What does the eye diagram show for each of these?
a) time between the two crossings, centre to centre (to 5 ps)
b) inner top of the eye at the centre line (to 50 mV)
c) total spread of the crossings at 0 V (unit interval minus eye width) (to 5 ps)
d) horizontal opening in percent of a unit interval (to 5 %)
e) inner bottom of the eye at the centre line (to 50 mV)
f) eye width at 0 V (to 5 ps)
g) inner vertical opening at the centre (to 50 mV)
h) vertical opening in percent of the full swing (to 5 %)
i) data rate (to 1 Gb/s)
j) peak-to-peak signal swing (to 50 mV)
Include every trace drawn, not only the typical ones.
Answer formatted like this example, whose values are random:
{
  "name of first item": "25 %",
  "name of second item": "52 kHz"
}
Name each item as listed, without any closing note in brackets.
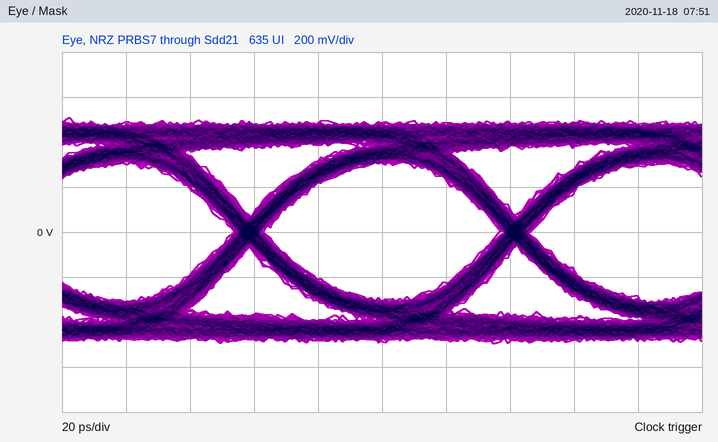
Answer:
{
  "time between the two crossings, centre to centre": "85 ps",
  "inner top of the eye at the centre line": "300 mV",
  "total spread of the crossings at 0 V (unit interval minus eye width)": "10 ps",
  "horizontal opening in percent of a unit interval": "90 %",
  "inner bottom of the eye at the centre line": "-300 mV",
  "eye width at 0 V": "75 ps",
  "inner vertical opening at the centre": "600 mV",
  "vertical opening in percent of the full swing": "60 %",
  "data rate": "12 Gb/s",
  "peak-to-peak signal swing": "1.00 V"
}
